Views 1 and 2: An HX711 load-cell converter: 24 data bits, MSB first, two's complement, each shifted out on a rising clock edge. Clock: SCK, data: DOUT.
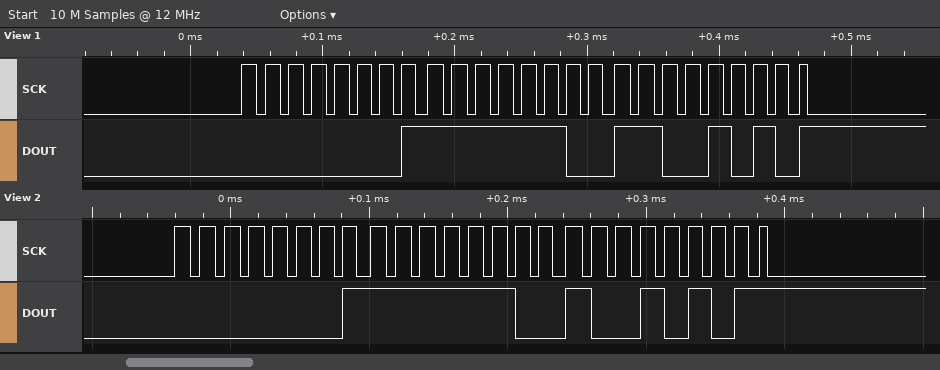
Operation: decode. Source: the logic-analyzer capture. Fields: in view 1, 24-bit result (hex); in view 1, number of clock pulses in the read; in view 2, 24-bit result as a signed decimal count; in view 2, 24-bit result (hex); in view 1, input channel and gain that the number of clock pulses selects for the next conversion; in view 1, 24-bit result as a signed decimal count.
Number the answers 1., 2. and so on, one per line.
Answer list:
1. 0x01FCCA
2. 25
3. 130197
4. 0x01FC95
5. channel A, gain 128
6. 130250
